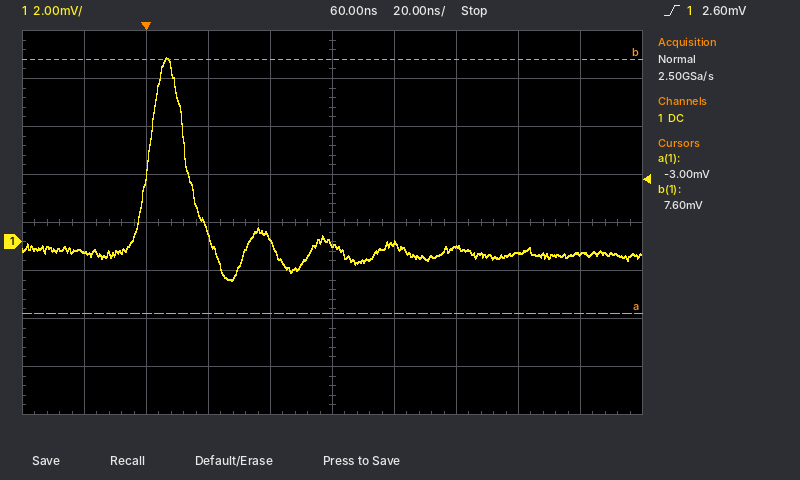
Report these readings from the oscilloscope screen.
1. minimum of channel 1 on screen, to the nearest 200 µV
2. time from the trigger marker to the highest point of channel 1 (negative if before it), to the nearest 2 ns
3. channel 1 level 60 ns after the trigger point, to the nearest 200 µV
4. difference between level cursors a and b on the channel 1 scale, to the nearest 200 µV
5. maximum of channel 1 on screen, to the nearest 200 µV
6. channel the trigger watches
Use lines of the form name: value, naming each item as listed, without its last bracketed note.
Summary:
minimum of channel 1 on screen, to the nearest 200 µV: -1.6 mV
time from the trigger marker to the highest point of channel 1 (negative if before it), to the nearest 2 ns: +6 ns
channel 1 level 60 ns after the trigger point, to the nearest 200 µV: 0.0 mV
difference between level cursors a and b on the channel 1 scale, to the nearest 200 µV: 10.6 mV
maximum of channel 1 on screen, to the nearest 200 µV: 7.6 mV
channel the trigger watches: channel 1
